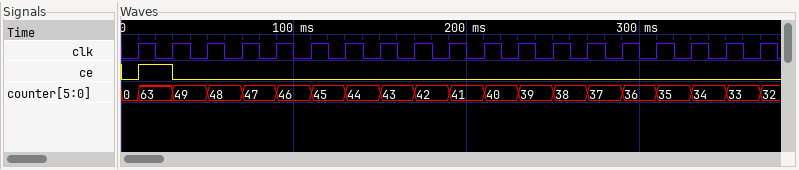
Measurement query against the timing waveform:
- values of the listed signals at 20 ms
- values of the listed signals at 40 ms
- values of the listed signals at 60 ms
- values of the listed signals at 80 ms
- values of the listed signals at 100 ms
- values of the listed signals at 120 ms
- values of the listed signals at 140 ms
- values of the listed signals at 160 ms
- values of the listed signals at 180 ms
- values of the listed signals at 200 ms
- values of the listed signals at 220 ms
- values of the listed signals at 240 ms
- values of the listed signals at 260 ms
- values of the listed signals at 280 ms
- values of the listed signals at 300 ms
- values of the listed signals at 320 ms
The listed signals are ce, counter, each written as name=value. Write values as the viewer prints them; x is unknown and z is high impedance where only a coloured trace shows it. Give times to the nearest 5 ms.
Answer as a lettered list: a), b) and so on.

a) ce=1, counter=63
b) ce=0, counter=49
c) ce=0, counter=48
d) ce=0, counter=47
e) ce=0, counter=46
f) ce=0, counter=45
g) ce=0, counter=44
h) ce=0, counter=43
i) ce=0, counter=42
j) ce=0, counter=41
k) ce=0, counter=40
l) ce=0, counter=39
m) ce=0, counter=38
n) ce=0, counter=37
o) ce=0, counter=36
p) ce=0, counter=35
